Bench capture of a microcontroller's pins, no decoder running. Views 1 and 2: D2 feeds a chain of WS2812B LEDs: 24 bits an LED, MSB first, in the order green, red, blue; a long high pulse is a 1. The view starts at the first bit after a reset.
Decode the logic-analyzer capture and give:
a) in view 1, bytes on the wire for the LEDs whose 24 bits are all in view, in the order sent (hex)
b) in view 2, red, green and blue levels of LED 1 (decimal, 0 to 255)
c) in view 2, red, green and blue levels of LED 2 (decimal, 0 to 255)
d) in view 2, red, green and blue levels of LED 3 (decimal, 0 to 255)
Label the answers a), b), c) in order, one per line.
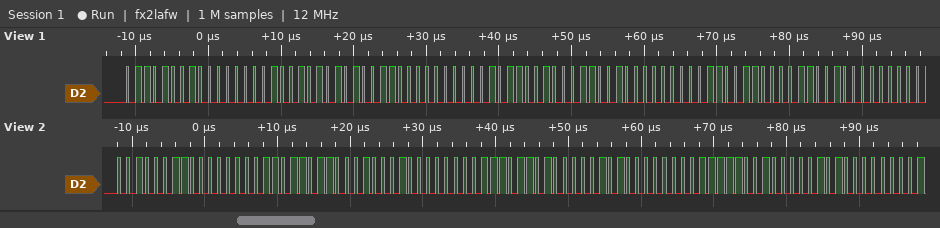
a) 69 00 95 4C 00 B2 32 00 CC
b) 0, 35, 219
c) 0, 17, 237
d) 0, 5, 249
